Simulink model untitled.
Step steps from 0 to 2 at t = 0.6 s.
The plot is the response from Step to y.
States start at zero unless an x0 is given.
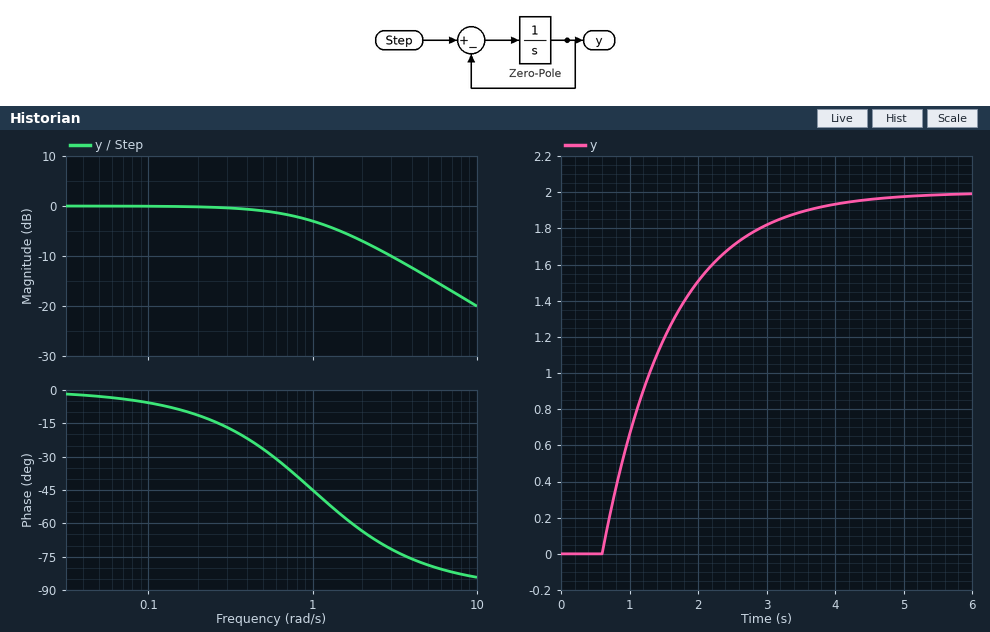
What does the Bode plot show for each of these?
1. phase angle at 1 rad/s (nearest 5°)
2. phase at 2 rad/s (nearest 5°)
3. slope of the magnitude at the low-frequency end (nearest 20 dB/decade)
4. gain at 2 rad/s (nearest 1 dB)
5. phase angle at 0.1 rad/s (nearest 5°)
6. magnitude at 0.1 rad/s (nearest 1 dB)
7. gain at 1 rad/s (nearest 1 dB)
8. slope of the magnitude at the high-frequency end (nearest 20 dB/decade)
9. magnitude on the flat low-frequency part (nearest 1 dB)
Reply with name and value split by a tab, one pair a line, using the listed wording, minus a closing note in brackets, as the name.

phase angle at 1 rad/s	-45°
phase at 2 rad/s	-65°
slope of the magnitude at the low-frequency end	0 dB/decade
gain at 2 rad/s	-7 dB
phase angle at 0.1 rad/s	-5°
magnitude at 0.1 rad/s	0 dB
gain at 1 rad/s	-3 dB
slope of the magnitude at the high-frequency end	-20 dB/decade
magnitude on the flat low-frequency part	0 dB
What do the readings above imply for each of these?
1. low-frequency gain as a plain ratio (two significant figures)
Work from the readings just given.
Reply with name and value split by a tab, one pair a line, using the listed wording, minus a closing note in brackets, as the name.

low-frequency gain as a plain ratio	1.0
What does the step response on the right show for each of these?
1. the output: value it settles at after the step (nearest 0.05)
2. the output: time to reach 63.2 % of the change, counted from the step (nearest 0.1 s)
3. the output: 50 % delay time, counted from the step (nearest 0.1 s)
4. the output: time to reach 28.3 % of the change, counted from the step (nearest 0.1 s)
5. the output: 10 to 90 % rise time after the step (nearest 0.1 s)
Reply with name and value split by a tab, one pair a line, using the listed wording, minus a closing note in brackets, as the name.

the output: value it settles at after the step	2.00
the output: time to reach 63.2 % of the change, counted from the step	1.0 s
the output: 50 % delay time, counted from the step	0.7 s
the output: time to reach 28.3 % of the change, counted from the step	0.3 s
the output: 10 to 90 % rise time after the step	2.2 s
